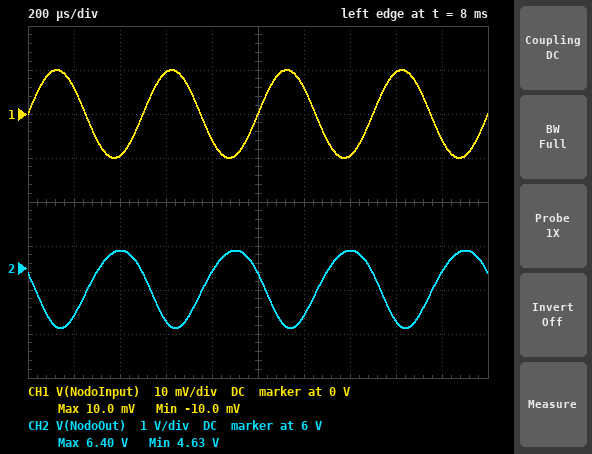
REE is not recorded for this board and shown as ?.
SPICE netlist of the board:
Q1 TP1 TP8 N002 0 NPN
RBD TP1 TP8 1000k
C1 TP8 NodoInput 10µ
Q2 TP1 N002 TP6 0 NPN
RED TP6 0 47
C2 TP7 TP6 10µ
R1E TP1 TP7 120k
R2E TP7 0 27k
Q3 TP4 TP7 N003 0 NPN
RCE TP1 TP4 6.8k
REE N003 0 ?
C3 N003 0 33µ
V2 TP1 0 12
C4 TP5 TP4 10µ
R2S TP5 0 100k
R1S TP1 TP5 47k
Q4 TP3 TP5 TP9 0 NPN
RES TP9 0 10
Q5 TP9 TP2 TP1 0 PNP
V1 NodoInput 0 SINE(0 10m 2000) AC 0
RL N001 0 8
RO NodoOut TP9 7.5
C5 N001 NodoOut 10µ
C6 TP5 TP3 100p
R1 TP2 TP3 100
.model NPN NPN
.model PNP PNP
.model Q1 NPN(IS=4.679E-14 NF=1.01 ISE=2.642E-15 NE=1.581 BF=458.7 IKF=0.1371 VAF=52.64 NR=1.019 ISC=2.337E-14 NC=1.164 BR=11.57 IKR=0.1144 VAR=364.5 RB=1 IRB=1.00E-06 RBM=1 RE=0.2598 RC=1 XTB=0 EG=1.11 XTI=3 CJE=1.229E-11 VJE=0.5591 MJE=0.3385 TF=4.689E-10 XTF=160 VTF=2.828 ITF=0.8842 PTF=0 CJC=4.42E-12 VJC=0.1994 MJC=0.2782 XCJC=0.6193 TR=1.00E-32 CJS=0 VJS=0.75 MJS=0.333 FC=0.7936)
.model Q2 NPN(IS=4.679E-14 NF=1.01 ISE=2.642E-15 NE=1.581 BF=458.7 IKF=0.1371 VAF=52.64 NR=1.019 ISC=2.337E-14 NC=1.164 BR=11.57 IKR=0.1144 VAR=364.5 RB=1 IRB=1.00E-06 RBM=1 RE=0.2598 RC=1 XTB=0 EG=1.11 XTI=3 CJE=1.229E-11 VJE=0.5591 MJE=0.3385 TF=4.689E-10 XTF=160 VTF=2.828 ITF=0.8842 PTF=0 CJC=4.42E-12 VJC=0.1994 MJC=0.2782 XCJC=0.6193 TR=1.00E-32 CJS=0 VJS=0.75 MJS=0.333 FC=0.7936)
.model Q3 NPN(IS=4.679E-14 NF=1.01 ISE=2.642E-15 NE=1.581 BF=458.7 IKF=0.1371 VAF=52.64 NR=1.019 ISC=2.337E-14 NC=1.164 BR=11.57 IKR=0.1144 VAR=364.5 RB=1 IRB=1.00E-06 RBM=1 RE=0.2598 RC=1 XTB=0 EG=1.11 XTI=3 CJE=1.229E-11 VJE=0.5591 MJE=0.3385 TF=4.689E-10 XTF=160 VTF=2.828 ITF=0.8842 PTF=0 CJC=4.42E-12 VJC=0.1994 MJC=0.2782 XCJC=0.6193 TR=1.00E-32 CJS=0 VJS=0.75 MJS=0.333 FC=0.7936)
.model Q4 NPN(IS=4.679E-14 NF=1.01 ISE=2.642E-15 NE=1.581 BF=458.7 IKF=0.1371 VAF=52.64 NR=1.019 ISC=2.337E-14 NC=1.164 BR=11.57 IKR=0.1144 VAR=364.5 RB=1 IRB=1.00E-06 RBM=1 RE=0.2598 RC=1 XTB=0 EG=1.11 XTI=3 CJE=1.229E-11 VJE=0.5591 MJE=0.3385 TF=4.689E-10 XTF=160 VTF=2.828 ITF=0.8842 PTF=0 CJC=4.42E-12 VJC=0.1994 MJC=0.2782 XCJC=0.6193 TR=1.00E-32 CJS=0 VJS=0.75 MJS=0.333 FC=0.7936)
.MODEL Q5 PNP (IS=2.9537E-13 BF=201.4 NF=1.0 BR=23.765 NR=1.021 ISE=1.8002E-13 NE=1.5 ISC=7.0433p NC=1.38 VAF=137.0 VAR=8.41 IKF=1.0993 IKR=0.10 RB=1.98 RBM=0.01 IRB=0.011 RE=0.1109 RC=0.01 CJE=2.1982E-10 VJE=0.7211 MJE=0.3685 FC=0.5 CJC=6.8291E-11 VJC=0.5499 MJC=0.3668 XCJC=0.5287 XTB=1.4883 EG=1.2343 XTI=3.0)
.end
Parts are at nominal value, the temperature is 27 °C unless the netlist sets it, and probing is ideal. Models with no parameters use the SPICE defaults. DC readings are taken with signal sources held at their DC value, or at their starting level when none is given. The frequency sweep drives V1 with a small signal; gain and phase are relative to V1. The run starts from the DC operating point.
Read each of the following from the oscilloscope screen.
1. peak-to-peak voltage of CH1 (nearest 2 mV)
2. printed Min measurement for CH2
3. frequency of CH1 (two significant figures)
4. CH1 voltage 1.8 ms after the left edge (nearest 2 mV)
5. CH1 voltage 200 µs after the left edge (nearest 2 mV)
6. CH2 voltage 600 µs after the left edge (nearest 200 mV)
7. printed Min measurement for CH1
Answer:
20 mV
4.63 V
2.0 kHz
-6 mV
6 mV
4.8 V
-10.0 mV
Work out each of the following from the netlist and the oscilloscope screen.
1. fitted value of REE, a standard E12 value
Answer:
1.8 kΩ
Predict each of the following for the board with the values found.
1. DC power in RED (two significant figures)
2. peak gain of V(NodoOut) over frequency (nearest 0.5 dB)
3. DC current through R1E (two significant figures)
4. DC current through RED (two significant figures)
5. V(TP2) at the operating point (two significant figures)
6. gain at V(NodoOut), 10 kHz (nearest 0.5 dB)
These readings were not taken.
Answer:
240 mW
42.0 dB
83 µA
71 mA
11 V
37.0 dB
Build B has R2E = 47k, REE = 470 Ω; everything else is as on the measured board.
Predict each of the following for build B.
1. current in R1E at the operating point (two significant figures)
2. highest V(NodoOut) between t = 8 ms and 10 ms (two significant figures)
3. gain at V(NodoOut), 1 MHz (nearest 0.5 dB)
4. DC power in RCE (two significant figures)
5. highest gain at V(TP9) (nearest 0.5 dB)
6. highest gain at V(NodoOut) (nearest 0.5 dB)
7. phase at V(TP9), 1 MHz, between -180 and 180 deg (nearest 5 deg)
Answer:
87 µA
7.9 V
20.0 dB
18 mW
26.0 dB
22.5 dB
165 deg
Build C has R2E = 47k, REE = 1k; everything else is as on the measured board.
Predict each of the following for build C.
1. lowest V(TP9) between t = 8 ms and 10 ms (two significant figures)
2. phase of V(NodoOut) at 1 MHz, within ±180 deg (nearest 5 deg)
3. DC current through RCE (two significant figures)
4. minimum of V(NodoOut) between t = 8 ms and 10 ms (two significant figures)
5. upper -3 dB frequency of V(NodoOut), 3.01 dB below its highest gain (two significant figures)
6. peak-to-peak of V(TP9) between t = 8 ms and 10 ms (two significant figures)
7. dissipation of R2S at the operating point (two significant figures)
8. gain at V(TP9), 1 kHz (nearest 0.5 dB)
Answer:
5.4 V
150 deg
1.5 mA
5.7 V
580 kHz
3.1 V
410 µW
31.0 dB
